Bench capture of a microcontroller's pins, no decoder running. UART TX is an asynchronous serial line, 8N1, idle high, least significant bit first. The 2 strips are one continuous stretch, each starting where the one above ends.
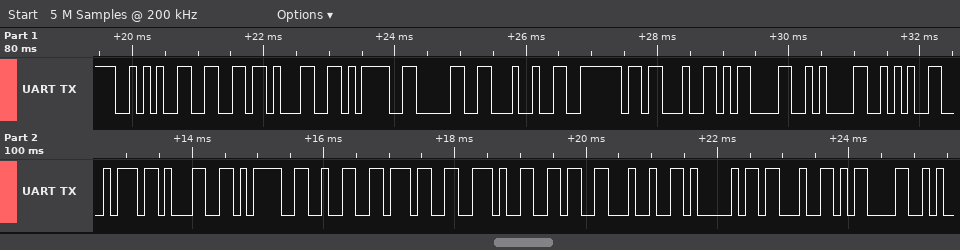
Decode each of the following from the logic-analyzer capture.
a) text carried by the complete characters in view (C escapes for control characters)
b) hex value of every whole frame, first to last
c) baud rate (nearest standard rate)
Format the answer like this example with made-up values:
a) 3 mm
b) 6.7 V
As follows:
a) "*f1=0$~#\r\n*t1=27.6$A#\r"
b) 2A 66 31 3D 30 24 7E 23 0D 0A 2A 74 31 3D 32 37 2E 36 24 41 23 0D
c) 9600 baud
